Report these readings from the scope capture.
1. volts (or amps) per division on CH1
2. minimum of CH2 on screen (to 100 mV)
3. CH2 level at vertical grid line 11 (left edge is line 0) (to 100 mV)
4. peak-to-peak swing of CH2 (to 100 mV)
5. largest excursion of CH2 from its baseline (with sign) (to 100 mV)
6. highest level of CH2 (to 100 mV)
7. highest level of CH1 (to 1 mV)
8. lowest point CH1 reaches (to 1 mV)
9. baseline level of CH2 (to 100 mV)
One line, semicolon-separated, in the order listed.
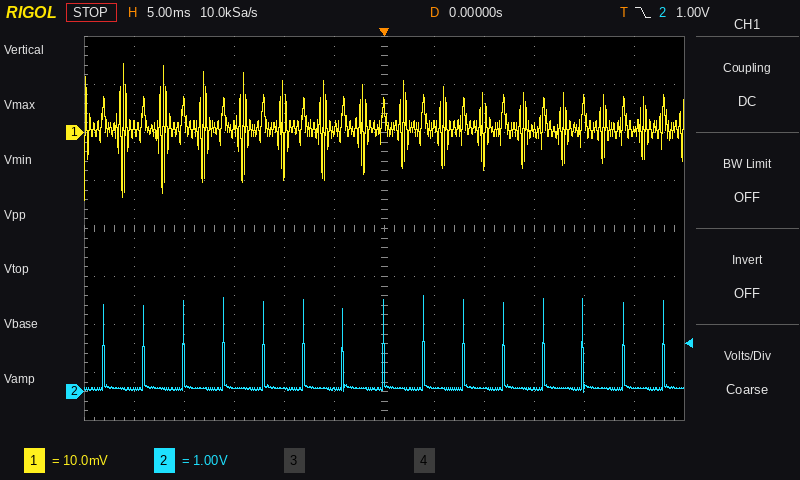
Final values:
10 mV; 0.0 V; 100 mV; 2.0 V; +1.9 V; 2.0 V; 14 mV; -14 mV; 100 mV
